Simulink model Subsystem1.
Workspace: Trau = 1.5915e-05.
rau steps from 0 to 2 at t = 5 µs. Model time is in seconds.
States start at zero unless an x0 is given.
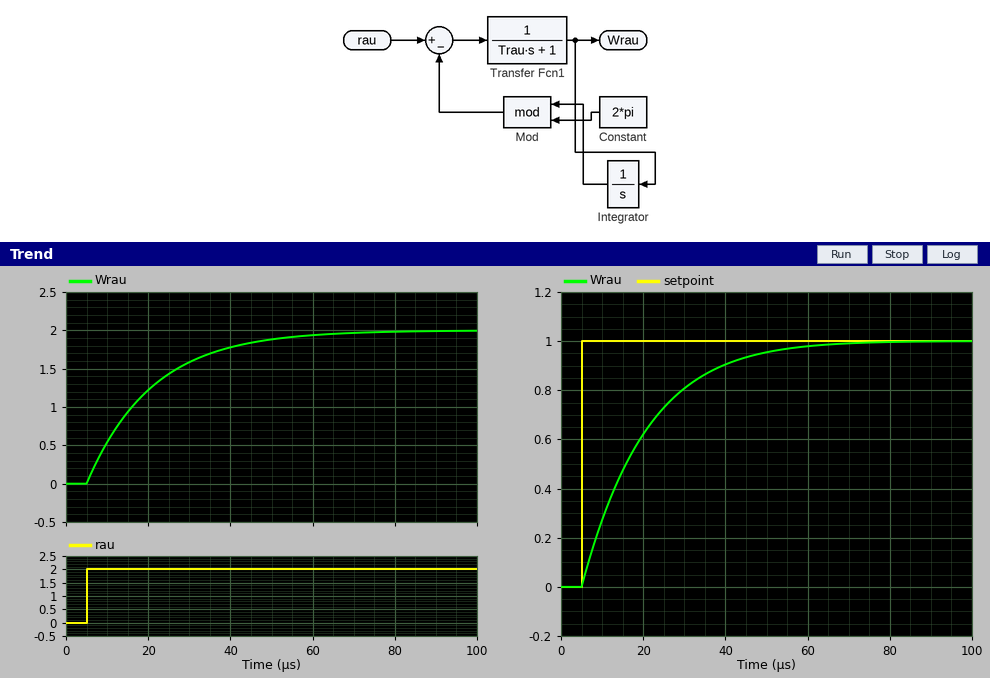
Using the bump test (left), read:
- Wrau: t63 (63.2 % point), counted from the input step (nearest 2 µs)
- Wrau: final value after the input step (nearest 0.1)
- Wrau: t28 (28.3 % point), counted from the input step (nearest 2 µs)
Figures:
16 µs
2.0
6 µs
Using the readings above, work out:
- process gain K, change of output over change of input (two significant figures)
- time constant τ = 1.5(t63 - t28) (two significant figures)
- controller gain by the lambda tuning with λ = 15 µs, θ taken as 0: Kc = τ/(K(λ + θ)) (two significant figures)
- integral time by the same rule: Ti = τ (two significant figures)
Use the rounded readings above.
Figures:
1.0
15 µs
1.0
15 µs
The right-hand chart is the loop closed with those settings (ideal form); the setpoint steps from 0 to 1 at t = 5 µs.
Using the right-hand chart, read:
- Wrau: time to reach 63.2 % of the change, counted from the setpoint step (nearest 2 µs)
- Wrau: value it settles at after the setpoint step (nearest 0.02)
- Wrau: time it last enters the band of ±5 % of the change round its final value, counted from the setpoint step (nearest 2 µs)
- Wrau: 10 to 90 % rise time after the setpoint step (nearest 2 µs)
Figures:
16 µs
1.00
44 µs
32 µs
